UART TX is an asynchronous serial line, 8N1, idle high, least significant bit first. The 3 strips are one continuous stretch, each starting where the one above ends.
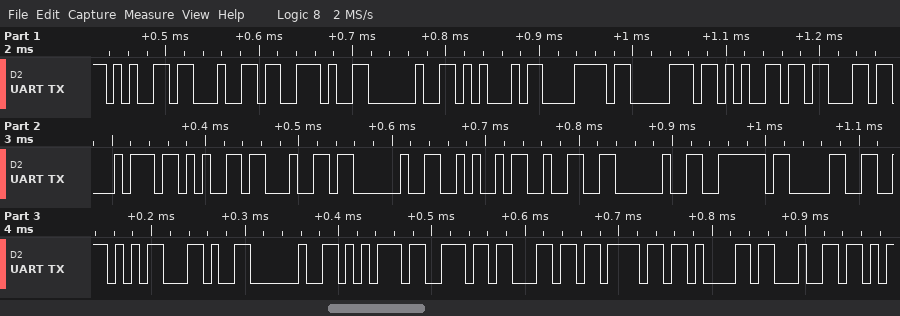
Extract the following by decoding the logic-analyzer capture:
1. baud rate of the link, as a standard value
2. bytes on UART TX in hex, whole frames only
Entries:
115200 baud
65 64 2E 20 45 78 70 65 63 74 65 64 20 4A 32 20 7E 30 56 2C 20 75 6E 6C 6F 61 64
